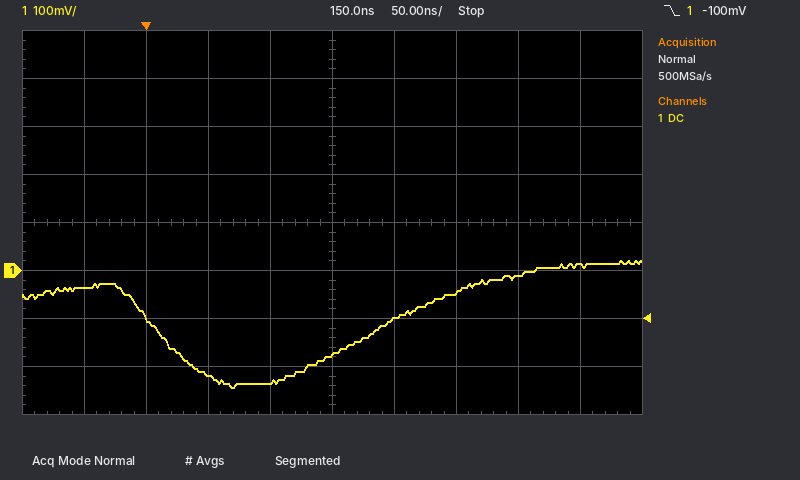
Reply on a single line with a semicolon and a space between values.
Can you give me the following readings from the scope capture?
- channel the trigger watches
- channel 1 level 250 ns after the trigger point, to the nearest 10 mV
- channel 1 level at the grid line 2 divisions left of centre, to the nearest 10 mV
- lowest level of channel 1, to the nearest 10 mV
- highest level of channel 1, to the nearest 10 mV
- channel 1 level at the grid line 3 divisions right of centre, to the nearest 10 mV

channel 1; -50 mV; -220 mV; -240 mV; 20 mV; -10 mV
